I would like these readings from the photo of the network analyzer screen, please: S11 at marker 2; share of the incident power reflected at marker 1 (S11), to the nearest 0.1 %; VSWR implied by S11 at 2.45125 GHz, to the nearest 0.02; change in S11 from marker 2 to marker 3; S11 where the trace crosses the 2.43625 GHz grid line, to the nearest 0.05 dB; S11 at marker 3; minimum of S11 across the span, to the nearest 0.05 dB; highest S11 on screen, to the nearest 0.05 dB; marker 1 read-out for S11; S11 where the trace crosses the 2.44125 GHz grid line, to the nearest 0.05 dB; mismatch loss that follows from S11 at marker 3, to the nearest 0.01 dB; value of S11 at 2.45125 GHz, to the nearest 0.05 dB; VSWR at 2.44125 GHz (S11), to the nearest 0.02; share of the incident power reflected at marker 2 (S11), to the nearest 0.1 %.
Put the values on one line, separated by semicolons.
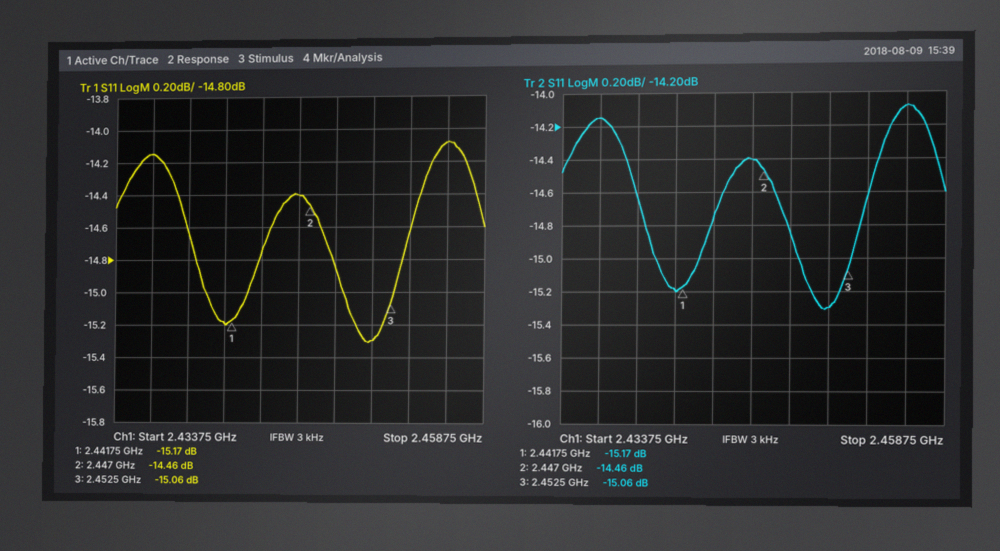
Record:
-14.46 dB; 3.0 %; 1.42; -0.60 dB; -14.15 dB; -15.06 dB; -15.30 dB; -14.10 dB; -15.17 dB; -15.20 dB; 0.14 dB; -15.30 dB; 1.42; 3.6 %
